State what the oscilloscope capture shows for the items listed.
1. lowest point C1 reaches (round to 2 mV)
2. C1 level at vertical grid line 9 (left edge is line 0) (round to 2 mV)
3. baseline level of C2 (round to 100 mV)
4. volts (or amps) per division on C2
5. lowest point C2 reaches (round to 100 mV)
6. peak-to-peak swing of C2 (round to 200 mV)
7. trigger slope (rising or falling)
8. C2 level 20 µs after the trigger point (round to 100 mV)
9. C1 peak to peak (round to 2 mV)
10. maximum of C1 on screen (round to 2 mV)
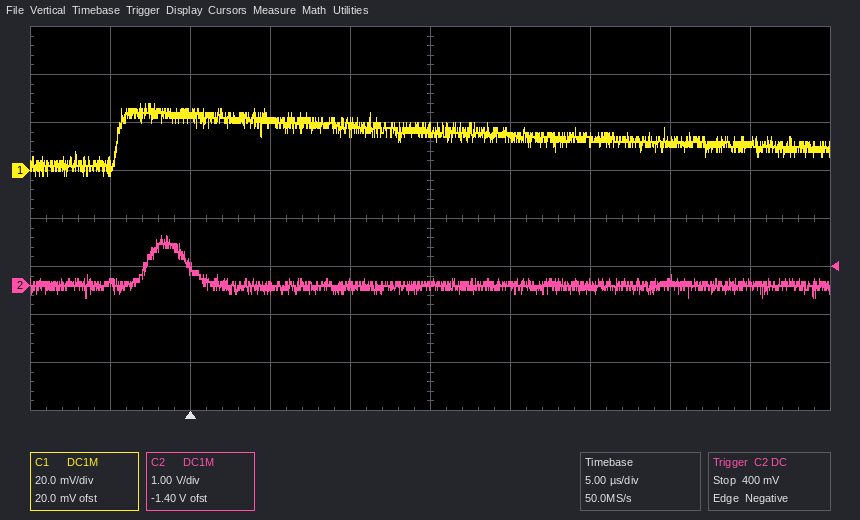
-2 mV
12 mV
0.0 V
1 V
-200 mV
1.2 V
falling
0.0 V
30 mV
28 mV
